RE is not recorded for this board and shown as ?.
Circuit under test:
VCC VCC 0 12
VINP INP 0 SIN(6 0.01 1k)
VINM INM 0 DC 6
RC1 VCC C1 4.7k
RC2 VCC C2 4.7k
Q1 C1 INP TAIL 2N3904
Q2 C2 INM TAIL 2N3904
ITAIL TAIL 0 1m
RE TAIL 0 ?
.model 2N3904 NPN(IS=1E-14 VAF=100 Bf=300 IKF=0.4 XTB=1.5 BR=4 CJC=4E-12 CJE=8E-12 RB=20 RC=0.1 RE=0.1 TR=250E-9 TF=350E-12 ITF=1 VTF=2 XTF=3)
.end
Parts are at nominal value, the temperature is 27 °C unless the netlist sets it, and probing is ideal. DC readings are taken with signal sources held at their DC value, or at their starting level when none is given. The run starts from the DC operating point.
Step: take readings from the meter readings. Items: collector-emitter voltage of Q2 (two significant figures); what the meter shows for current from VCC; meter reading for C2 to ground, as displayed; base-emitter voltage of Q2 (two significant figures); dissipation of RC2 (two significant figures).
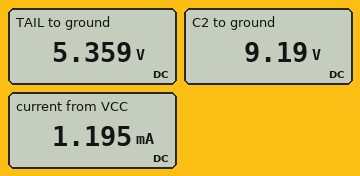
3.8 V
1.195 mA
9.19 V
640 mV
1.7 mW
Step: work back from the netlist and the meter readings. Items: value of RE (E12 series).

27 kΩ
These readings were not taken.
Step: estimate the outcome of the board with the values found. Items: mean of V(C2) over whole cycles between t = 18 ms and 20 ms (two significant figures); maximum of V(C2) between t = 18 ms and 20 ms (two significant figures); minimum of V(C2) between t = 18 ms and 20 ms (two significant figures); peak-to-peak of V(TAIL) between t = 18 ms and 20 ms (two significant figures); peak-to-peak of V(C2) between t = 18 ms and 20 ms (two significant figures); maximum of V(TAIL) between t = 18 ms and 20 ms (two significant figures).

9.2 V
9.7 V
8.7 V
10 mV
1.0 V
5.4 V
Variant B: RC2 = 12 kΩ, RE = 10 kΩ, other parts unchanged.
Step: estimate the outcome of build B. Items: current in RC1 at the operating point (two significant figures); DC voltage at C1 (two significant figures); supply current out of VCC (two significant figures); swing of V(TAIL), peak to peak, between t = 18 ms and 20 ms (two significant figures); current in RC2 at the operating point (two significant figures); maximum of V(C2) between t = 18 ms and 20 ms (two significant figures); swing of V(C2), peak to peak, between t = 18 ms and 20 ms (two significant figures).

920 µA
7.7 V
1.5 mA
17 mV
550 µA
5.4 V
51 mV
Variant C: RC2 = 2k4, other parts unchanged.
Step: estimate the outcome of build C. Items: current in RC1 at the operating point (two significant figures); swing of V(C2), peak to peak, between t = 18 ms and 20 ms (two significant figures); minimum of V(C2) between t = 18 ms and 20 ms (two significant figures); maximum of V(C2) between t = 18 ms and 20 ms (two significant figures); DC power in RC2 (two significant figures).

590 µA
530 mV
10 V
11 V
870 µW
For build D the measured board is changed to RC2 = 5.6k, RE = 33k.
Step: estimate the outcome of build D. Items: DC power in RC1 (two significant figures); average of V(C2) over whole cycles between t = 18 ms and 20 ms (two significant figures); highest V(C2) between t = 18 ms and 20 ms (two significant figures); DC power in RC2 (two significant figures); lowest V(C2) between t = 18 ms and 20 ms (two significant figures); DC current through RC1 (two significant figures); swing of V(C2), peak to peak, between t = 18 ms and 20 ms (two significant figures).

1.6 mW
8.8 V
9.4 V
1.9 mW
8.2 V
580 µA
1.2 V
